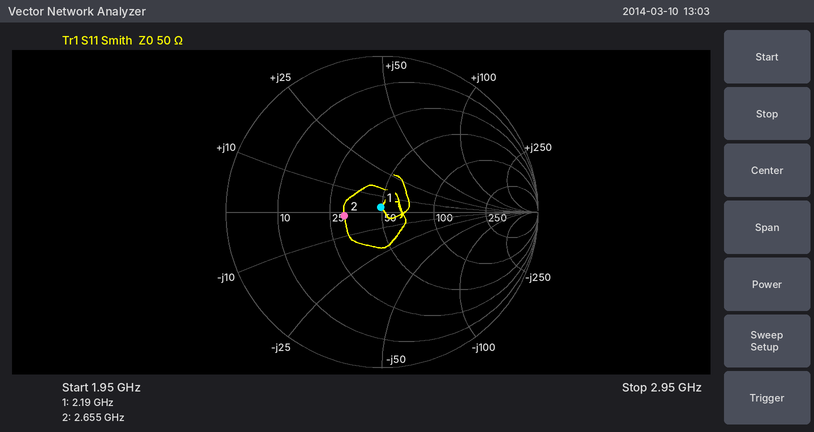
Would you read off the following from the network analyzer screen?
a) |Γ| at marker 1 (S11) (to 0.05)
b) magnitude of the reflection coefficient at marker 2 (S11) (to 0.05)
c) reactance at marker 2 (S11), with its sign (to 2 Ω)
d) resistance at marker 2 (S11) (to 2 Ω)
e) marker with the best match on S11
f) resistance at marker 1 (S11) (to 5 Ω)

0.05
0.25
-2 Ω
30 Ω
marker 1
50 Ω
